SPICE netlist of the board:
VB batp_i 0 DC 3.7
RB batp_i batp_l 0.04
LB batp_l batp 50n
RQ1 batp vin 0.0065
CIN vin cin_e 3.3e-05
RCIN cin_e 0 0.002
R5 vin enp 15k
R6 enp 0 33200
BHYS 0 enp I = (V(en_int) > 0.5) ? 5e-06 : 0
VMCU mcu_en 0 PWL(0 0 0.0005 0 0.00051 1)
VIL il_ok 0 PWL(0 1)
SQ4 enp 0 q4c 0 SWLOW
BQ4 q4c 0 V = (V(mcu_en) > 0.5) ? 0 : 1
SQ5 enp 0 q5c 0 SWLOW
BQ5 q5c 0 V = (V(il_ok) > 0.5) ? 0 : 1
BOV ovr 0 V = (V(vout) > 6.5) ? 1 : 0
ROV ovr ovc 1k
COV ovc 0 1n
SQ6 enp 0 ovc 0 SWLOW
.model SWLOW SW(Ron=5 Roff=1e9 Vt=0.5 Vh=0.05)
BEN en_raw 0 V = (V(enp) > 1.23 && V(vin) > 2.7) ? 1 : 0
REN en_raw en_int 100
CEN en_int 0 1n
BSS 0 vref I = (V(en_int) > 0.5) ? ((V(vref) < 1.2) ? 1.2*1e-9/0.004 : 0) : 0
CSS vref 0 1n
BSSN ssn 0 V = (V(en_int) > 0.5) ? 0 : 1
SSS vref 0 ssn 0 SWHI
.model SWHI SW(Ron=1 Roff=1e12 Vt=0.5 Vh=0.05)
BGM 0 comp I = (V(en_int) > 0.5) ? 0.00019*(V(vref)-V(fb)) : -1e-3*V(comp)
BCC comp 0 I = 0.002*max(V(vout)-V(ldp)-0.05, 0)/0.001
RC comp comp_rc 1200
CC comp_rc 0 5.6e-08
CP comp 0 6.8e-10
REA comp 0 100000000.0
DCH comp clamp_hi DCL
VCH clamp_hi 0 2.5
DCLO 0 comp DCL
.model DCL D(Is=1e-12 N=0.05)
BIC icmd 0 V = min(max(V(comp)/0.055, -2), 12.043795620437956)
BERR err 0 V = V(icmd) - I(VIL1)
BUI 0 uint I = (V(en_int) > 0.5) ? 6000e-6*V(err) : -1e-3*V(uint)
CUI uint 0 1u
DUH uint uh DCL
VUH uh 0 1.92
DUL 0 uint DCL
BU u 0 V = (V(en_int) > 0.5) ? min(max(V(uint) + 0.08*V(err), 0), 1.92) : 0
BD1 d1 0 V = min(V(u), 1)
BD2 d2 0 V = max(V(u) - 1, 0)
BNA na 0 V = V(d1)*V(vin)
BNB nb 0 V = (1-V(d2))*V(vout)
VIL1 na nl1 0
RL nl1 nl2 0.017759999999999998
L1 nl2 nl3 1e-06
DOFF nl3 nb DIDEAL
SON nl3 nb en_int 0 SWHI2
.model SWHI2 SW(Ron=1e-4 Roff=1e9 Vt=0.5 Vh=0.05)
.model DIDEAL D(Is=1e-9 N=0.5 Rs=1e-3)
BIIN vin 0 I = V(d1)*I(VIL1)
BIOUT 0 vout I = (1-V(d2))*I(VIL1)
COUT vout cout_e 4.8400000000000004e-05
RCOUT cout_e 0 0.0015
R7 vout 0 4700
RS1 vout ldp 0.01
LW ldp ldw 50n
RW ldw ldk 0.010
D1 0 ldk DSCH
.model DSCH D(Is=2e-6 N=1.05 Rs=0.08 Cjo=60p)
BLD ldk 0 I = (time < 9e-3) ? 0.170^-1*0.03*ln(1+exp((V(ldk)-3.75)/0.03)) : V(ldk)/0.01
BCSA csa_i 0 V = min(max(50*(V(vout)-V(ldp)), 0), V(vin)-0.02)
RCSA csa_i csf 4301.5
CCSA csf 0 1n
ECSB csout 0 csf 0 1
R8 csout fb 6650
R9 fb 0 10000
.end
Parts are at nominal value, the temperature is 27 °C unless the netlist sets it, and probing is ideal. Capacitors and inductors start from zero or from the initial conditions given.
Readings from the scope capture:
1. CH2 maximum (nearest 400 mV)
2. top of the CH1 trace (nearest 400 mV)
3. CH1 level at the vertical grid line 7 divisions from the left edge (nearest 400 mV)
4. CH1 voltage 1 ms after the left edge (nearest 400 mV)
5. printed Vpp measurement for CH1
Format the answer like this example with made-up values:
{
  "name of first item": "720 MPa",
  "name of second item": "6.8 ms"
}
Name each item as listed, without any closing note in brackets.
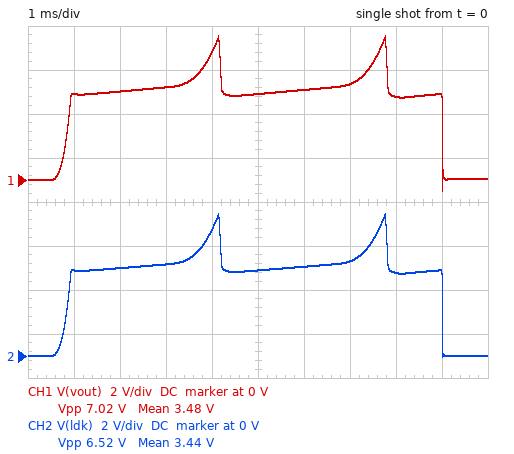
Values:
{
  "CH2 maximum": "6.4 V",
  "top of the CH1 trace": "6.4 V",
  "CH1 level at the vertical grid line 7 divisions from the left edge": "4.4 V",
  "CH1 voltage 1 ms after the left edge": "4.0 V",
  "printed Vpp measurement for CH1": "7.02 V"
}
